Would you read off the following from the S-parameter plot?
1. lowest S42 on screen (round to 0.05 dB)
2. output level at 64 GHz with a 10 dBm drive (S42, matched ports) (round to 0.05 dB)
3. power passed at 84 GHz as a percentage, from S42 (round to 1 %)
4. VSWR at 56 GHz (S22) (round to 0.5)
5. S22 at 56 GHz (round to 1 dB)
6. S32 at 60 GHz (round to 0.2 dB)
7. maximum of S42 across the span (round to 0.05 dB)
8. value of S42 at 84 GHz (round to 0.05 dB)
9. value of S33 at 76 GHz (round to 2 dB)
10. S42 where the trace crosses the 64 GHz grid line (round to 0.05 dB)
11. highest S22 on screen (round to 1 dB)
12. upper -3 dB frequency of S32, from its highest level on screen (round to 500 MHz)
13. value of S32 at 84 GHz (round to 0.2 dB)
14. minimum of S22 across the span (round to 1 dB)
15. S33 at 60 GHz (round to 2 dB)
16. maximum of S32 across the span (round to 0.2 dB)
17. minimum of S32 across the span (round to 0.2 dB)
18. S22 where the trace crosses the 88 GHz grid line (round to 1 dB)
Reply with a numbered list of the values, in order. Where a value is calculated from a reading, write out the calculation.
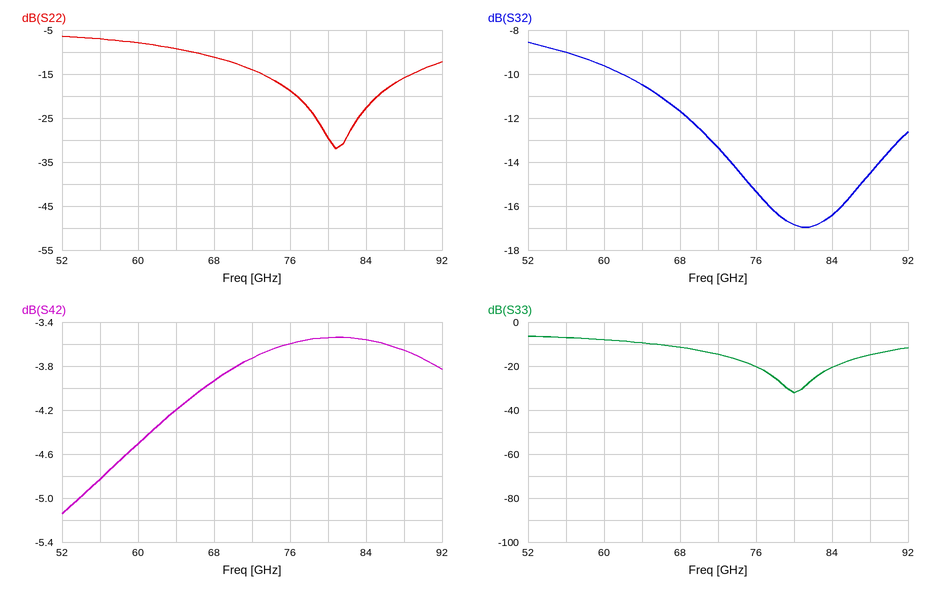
1. -5.15 dB
2. 10 dBm + (-4.20 dB) = 5.80 dBm
3. 10^(-3.55/10) ≈ 44 %
4. |Γ| = 10^(-7/20) = 0.4467; VSWR = (1 + 0.4467)/(1 − 0.4467) ≈ 2.61, so 2.5 to the nearest 0.5
5. -7 dB
6. -9.6 dB
7. -3.55 dB
8. -3.55 dB
9. -20 dB
10. -4.20 dB
11. -6 dB
12. 67.5 GHz
13. -16.4 dB
14. -32 dB
15. -8 dB
16. -8.6 dB
17. -17.0 dB
18. -16 dB
